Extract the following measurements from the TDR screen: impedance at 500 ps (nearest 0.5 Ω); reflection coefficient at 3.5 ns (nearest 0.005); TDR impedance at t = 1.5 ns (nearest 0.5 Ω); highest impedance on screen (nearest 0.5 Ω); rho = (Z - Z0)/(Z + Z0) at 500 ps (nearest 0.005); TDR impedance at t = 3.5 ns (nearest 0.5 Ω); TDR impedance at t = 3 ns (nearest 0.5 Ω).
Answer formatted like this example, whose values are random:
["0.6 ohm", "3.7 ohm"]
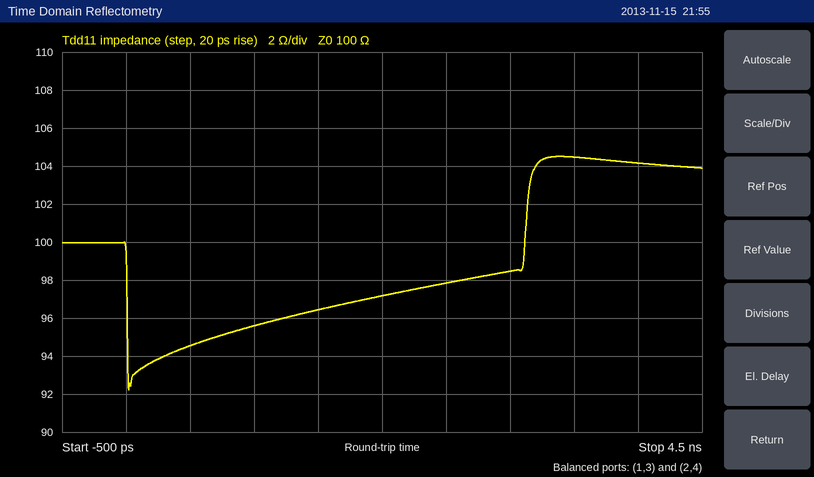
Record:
["94.5 Ω", "+0.020", "96.5 Ω", "104.5 Ω", "-0.030", "104.5 Ω", "98.5 Ω"]
